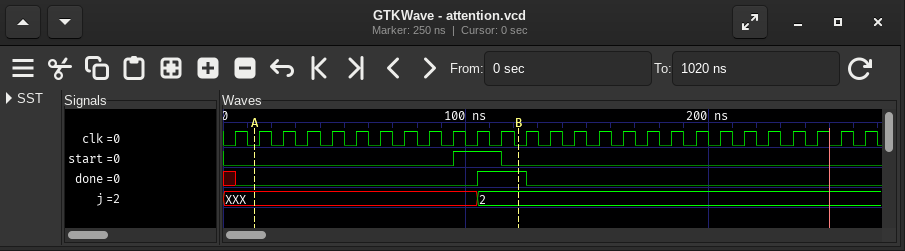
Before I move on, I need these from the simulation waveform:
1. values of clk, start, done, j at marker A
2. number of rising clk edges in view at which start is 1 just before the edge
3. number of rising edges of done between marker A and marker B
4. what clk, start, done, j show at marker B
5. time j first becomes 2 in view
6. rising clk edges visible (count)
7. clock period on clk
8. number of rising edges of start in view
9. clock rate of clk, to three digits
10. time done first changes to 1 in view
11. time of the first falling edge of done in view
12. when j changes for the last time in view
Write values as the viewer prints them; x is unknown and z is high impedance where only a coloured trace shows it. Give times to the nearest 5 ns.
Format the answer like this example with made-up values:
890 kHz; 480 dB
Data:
clk=0, start=0, done=0, j=XXX; 2; 1; clk=0, start=0, done=1, j=2; 105 ns; 27; 10 ns; 1; 100 MHz; 105 ns; 125 ns; 105 ns
